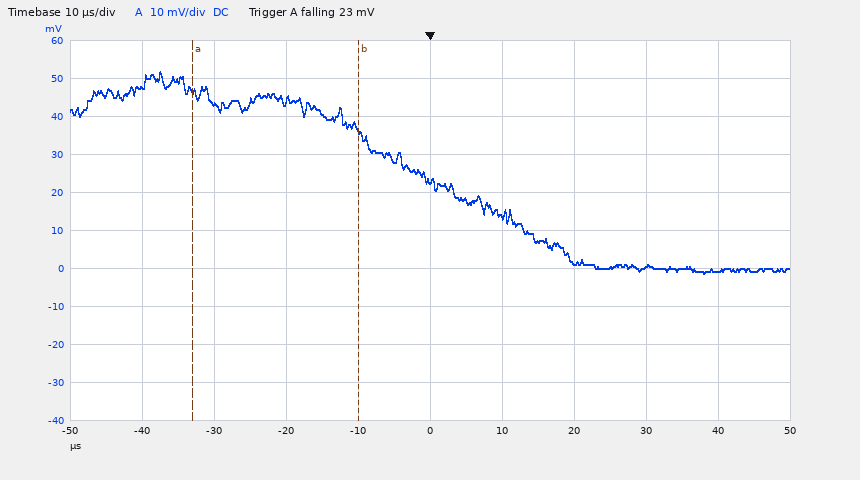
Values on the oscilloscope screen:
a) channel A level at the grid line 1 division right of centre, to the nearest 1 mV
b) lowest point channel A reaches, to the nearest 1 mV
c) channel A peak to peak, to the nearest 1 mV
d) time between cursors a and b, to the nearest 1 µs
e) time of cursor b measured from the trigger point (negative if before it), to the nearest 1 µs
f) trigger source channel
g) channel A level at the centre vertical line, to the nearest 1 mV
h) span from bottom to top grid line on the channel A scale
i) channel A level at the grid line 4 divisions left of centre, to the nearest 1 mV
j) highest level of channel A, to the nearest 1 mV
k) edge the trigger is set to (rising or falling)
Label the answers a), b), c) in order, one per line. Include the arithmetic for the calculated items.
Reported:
a) 14 mV
b) -1 mV
c) 52 mV − (-1 mV) = 53 mV
d) 23 µs
e) -10 µs
f) channel A
g) 23 mV
h) 100 mV
i) 48 mV
j) 52 mV
k) falling
